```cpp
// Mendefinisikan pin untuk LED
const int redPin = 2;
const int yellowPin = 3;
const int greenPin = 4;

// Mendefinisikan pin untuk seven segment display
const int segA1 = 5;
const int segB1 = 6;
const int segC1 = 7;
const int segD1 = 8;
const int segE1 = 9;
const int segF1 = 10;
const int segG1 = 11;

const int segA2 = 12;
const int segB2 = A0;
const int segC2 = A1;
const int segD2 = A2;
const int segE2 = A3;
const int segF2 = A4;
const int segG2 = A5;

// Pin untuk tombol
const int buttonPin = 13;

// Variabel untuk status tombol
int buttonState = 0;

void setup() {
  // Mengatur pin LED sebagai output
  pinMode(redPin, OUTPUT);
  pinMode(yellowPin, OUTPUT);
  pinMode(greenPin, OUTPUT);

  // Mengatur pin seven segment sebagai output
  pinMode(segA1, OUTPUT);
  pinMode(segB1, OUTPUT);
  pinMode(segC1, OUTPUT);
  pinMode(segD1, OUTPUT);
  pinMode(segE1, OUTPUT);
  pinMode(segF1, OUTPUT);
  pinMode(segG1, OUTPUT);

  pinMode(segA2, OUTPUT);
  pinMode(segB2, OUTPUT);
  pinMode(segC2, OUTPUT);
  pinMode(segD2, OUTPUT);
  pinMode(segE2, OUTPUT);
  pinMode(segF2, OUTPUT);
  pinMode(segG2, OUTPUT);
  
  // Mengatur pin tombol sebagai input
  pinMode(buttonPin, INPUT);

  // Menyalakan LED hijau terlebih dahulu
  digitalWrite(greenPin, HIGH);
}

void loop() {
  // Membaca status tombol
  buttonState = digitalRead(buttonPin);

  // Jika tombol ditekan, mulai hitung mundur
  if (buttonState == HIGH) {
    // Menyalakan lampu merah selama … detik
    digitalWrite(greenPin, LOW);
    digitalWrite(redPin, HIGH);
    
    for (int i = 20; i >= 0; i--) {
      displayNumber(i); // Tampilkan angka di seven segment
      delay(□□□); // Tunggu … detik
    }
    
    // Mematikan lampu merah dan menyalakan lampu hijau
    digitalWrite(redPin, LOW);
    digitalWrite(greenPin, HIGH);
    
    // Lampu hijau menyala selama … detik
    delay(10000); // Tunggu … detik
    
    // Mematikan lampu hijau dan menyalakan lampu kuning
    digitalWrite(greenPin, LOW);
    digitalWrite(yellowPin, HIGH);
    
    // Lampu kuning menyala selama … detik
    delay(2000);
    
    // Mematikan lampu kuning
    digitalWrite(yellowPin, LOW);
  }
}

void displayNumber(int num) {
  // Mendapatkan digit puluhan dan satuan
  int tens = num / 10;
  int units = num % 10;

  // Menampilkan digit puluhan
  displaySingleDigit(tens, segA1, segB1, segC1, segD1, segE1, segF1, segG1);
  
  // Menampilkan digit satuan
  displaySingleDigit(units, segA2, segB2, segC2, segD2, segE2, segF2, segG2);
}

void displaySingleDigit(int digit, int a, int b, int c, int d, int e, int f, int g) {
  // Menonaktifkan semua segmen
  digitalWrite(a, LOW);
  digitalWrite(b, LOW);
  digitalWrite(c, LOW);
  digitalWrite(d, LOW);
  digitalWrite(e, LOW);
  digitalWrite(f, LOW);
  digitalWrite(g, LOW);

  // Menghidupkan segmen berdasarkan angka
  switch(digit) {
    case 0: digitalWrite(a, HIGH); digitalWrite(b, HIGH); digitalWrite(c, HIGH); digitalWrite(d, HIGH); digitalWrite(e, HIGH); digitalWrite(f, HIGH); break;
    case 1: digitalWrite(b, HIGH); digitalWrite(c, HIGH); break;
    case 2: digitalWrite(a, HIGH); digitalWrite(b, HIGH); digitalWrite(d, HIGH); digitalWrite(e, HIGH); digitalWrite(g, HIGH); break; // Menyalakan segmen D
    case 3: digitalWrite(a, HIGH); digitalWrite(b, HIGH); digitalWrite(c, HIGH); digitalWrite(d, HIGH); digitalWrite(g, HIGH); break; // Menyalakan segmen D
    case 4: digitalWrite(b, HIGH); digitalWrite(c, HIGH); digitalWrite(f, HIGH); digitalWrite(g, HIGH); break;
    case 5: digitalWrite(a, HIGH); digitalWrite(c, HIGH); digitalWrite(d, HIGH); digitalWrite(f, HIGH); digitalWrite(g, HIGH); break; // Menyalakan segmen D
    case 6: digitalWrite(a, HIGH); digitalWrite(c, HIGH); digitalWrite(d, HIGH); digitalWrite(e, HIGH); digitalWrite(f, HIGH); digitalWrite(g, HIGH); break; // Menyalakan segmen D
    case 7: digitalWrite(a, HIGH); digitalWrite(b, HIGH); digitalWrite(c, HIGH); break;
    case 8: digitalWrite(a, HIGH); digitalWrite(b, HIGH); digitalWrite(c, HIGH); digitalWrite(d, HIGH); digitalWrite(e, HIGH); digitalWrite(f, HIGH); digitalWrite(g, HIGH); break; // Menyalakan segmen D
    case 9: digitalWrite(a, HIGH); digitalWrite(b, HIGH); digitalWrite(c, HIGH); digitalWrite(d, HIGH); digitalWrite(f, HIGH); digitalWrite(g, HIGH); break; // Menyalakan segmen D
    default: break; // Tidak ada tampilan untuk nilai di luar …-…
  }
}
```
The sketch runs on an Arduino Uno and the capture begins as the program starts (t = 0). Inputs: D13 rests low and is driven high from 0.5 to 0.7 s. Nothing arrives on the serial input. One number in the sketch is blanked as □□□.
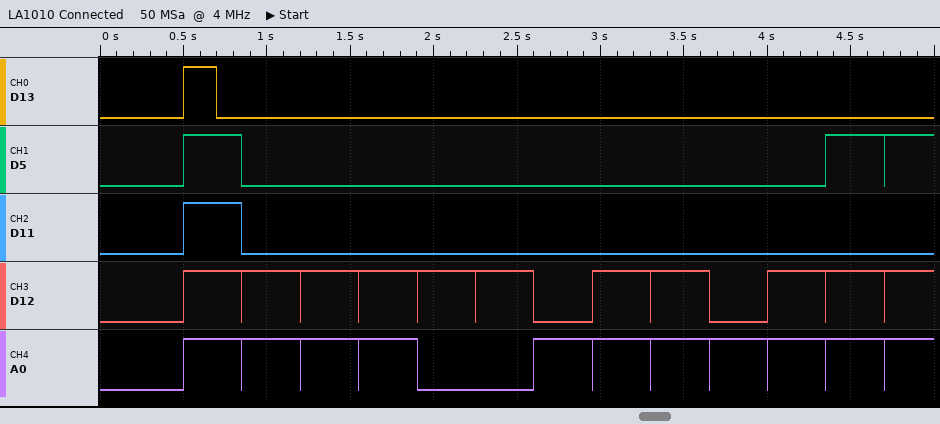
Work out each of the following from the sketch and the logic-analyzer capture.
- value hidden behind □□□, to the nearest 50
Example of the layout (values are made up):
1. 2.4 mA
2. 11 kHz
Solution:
1. 350
